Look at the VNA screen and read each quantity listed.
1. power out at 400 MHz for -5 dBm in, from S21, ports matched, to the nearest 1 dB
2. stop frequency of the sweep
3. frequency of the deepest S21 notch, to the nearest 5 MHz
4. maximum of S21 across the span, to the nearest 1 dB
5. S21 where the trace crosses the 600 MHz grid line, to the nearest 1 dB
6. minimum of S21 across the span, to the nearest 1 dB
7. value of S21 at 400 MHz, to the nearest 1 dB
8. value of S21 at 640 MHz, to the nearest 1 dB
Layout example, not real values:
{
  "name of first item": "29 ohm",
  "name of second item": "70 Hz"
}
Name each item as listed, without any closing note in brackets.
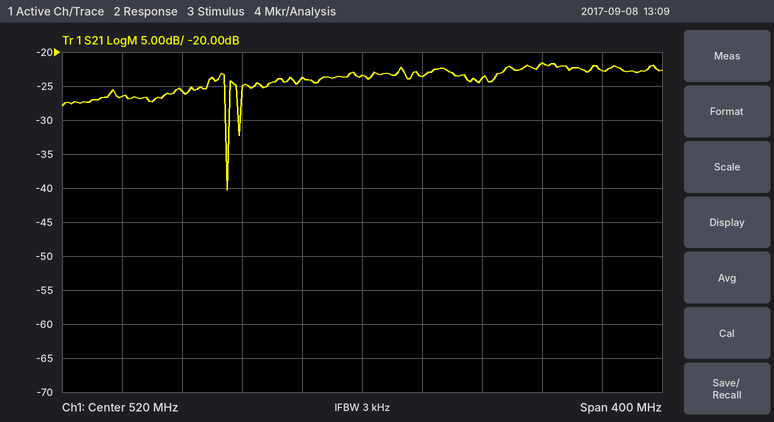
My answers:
{
  "power out at 400 MHz for -5 dBm in, from S21, ports matched, to the nearest 1 dB": "-31 dBm",
  "stop frequency of the sweep": "720 MHz",
  "frequency of the deepest S21 notch, to the nearest 5 MHz": "430 MHz",
  "maximum of S21 across the span, to the nearest 1 dB": "-22 dB",
  "S21 where the trace crosses the 600 MHz grid line, to the nearest 1 dB": "-24 dB",
  "minimum of S21 across the span, to the nearest 1 dB": "-40 dB",
  "value of S21 at 400 MHz, to the nearest 1 dB": "-26 dB",
  "value of S21 at 640 MHz, to the nearest 1 dB": "-22 dB"
}
